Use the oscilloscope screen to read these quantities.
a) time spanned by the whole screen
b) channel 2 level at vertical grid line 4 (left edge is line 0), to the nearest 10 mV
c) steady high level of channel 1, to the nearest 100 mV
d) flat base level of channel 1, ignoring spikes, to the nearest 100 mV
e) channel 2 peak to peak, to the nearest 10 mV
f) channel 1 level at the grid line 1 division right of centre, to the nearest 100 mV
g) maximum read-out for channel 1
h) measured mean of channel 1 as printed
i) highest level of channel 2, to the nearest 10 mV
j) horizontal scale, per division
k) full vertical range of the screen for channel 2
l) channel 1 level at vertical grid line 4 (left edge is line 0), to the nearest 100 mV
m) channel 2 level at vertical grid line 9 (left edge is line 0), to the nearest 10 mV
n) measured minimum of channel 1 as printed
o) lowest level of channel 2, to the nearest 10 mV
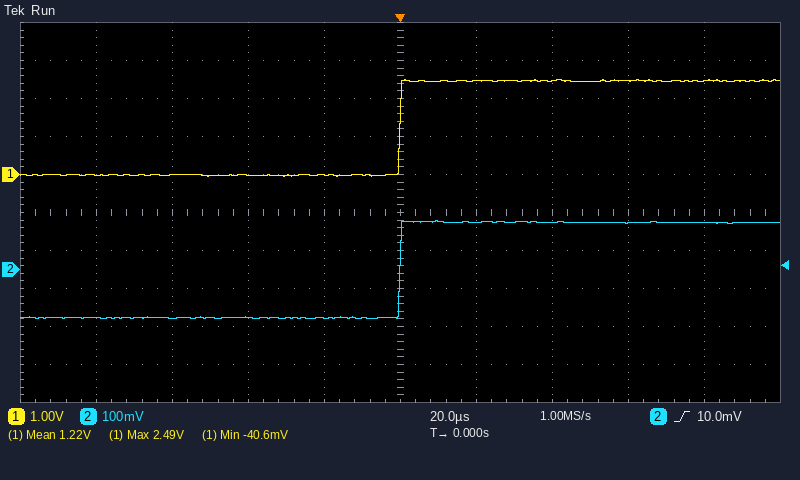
200 µs
-130 mV
2.5 V
0.0 V
260 mV
2.5 V
2.49 V
1.22 V
130 mV
20 µs
1 V
0.0 V
120 mV
-40.6 mV
-130 mV
